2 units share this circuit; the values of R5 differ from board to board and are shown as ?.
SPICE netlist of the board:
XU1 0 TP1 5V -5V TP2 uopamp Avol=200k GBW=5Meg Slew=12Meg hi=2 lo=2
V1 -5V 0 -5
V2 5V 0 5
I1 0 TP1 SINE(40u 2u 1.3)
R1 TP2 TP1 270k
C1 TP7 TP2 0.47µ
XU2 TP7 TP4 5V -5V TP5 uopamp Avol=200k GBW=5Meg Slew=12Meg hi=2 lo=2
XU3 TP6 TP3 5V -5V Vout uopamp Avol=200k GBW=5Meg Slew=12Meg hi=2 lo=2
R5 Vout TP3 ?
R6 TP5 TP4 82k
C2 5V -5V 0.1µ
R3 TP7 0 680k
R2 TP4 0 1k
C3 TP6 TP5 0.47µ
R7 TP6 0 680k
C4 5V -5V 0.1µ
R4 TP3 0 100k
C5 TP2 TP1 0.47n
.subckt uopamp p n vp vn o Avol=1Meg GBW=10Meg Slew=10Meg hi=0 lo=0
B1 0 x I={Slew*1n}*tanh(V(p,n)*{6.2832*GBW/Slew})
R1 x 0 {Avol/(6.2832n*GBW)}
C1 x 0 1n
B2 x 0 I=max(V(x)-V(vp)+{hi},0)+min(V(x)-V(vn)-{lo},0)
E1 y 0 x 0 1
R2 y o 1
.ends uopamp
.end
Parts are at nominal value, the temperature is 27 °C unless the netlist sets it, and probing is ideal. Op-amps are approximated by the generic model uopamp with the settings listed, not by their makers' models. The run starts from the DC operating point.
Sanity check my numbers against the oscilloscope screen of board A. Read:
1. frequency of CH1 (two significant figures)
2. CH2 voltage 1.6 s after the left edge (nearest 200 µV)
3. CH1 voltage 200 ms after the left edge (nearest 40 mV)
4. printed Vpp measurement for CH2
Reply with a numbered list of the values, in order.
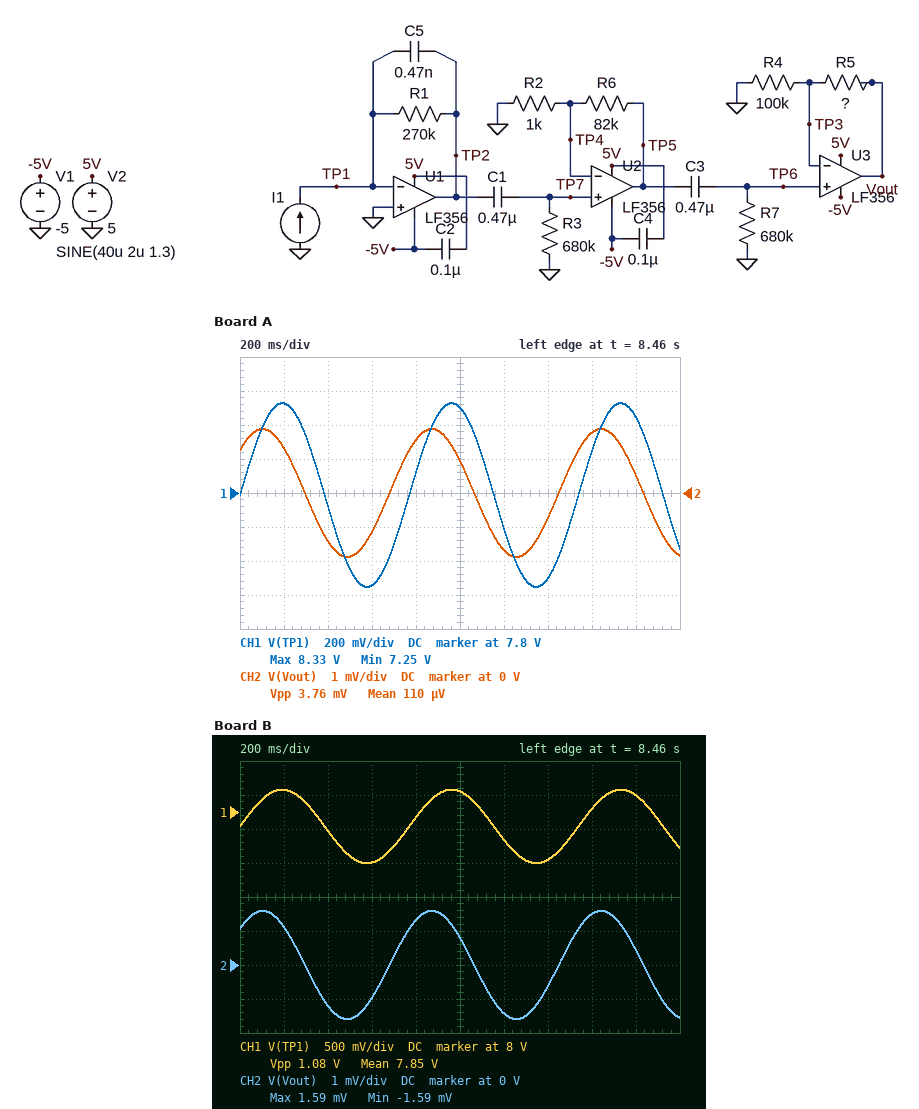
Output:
1. 1.3 Hz
2. 1.8 mV
3. 8.32 V
4. 3.76 mV
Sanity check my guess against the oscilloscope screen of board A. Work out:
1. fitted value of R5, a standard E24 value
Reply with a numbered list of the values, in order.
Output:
1. 1.2 MΩ
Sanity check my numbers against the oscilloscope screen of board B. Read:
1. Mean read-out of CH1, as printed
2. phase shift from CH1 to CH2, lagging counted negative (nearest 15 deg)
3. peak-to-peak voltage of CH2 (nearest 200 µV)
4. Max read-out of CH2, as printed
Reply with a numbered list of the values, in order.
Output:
1. 7.85 V
2. 45 deg
3. 3.2 mV
4. 1.59 mV
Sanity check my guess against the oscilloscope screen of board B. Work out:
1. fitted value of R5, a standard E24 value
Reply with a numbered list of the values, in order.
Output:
1. 1 MΩ
